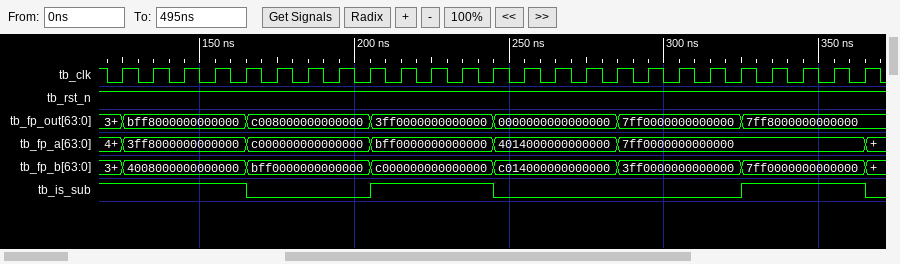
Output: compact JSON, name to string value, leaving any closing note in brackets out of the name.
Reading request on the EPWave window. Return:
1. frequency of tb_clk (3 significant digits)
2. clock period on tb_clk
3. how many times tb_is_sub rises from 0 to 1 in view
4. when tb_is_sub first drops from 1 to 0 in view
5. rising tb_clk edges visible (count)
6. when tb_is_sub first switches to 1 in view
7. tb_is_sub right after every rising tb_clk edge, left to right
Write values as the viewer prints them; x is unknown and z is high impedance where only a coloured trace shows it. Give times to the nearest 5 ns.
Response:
{"frequency of tb_clk": "100 MHz", "clock period on tb_clk": "10 ns", "how many times tb_is_sub rises from 0 to 1 in view": "2", "when tb_is_sub first drops from 1 to 0 in view": "165 ns", "rising tb_clk edges visible": "25", "when tb_is_sub first switches to 1 in view": "205 ns", "tb_is_sub right after every rising tb_clk edge, left to right": "1 1 1 1 0 0 0 0 1 1 1 1 0 0 0 0 0 0 0 0 1 1 1 1 0"}
